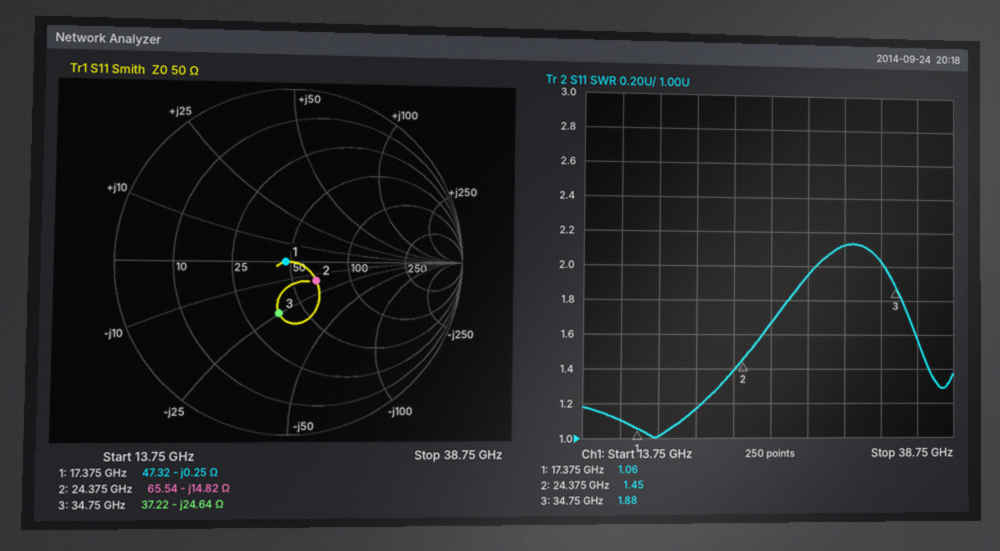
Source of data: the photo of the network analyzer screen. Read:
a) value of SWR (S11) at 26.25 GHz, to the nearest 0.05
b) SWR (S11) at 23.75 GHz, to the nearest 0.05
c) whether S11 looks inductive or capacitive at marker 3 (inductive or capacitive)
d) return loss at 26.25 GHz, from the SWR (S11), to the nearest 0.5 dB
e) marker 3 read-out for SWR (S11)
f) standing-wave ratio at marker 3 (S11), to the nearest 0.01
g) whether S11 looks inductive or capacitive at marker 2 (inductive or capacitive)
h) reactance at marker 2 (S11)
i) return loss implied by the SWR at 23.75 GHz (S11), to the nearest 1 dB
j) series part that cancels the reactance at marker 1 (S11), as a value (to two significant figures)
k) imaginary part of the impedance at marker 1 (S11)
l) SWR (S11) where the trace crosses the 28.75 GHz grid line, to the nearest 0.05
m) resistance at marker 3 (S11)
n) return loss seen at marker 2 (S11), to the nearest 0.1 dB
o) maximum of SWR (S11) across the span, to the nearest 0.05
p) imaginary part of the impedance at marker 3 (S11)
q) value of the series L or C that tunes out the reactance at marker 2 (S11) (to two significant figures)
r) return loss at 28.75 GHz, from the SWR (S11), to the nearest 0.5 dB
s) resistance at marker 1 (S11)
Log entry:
1.65
1.40
capacitive
12.0 dB
1.88
1.88
capacitive
-14.82 Ω
16 dB
2.3 pH
-0.25 Ω
1.95
37.22 Ω
14.7 dB
2.15
-24.64 Ω
97 pH
10.0 dB
47.32 Ω
